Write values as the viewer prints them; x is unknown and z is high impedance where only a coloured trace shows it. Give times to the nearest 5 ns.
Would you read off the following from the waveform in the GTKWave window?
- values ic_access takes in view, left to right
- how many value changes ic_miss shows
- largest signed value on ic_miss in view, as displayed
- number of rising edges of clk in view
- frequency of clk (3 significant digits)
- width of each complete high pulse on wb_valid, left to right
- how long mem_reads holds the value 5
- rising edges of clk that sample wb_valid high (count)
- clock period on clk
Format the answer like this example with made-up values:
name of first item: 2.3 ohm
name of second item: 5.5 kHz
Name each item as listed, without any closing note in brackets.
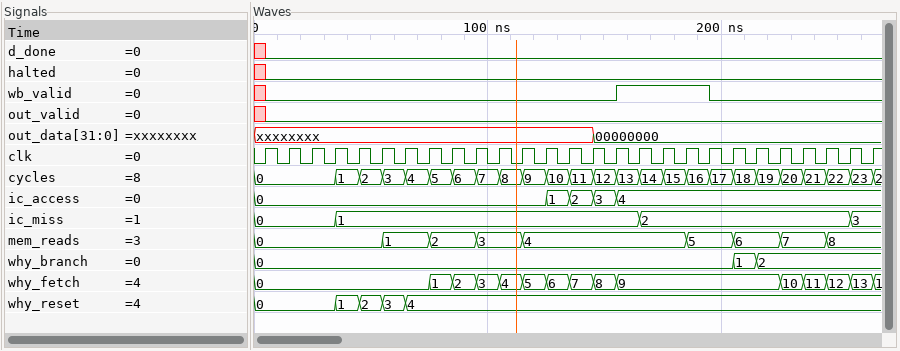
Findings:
values ic_access takes in view, left to right: 0, 1, 2, 3, 4
how many value changes ic_miss shows: 3
largest signed value on ic_miss in view, as displayed: 3
number of rising edges of clk in view: 27
frequency of clk: 100 MHz
width of each complete high pulse on wb_valid, left to right: 40 ns
how long mem_reads holds the value 5: 20 ns
rising edges of clk that sample wb_valid high: 4
clock period on clk: 10 ns
